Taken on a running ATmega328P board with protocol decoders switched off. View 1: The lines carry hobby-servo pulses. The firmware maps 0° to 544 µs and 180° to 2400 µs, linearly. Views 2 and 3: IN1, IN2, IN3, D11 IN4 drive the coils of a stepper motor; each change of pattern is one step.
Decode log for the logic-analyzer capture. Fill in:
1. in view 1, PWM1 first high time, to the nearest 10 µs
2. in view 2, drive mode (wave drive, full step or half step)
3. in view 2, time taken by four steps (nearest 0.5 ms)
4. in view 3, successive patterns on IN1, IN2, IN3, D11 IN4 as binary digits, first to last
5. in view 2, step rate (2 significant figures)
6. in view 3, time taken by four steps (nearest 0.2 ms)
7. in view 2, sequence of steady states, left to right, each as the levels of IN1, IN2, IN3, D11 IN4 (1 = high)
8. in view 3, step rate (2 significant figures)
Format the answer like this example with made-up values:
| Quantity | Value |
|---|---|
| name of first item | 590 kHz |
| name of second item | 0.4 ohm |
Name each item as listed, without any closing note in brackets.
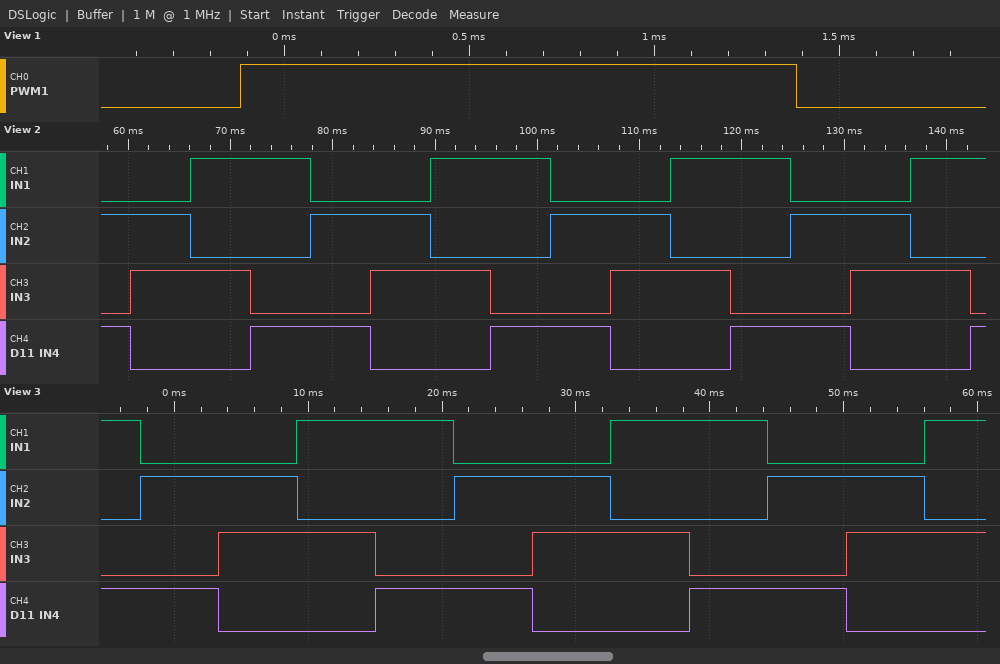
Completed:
| Quantity | Value |
|---|---|
| in view 1, PWM1 first high time, to the nearest 10 µs | 1500 µs |
| in view 2, drive mode | full step |
| in view 2, time taken by four steps | 23.5 ms |
| in view 3, successive patterns on IN1, IN2, IN3, D11 IN4 as binary digits, first to last | 1001 0101 0110 1010 1001 0101 0110 1010 1001 0101 0110 1010 |
| in view 2, step rate | 170 steps/s |
| in view 3, time taken by four steps | 23.4 ms |
| in view 2, sequence of steady states, left to right, each as the levels of IN1, IN2, IN3, D11 IN4 | 0101 0110 1010 1001 0101 0110 1010 1001 0101 0110 1010 1001 0101 0110 1010 1001 |
| in view 3, step rate | 170 steps/s |
